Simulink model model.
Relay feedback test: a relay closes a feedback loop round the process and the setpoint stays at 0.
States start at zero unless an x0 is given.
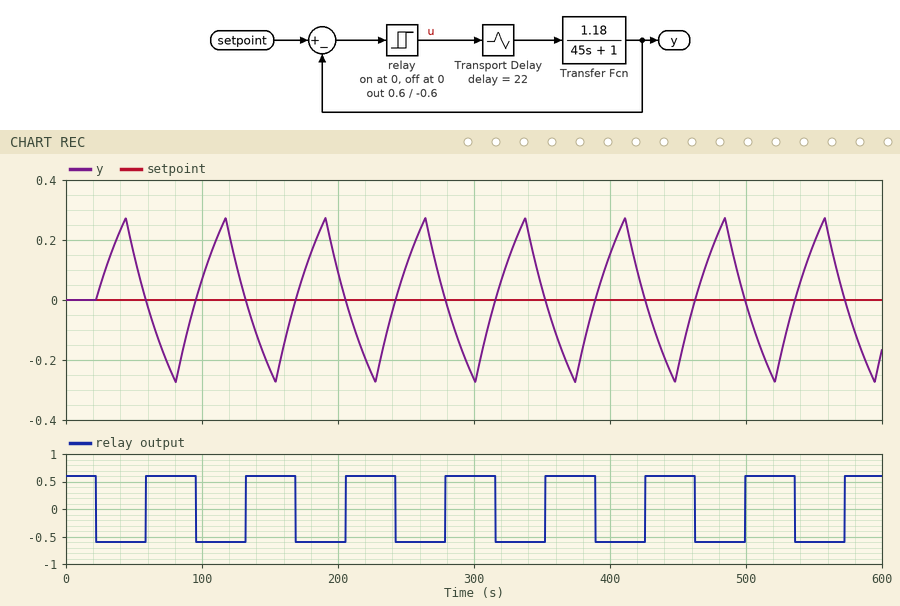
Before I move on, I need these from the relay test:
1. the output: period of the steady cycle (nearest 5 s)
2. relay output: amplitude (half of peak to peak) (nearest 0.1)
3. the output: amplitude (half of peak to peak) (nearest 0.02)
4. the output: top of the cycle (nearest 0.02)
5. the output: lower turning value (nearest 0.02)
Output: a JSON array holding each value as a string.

["75 s", "0.6", "0.28", "0.28", "-0.28"]
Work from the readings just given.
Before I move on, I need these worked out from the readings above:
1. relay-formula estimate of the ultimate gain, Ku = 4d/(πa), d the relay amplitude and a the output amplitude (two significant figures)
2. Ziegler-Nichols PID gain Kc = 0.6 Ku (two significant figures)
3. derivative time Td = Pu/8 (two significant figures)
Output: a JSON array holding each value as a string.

["2.7", "1.6", "9.4 s"]
